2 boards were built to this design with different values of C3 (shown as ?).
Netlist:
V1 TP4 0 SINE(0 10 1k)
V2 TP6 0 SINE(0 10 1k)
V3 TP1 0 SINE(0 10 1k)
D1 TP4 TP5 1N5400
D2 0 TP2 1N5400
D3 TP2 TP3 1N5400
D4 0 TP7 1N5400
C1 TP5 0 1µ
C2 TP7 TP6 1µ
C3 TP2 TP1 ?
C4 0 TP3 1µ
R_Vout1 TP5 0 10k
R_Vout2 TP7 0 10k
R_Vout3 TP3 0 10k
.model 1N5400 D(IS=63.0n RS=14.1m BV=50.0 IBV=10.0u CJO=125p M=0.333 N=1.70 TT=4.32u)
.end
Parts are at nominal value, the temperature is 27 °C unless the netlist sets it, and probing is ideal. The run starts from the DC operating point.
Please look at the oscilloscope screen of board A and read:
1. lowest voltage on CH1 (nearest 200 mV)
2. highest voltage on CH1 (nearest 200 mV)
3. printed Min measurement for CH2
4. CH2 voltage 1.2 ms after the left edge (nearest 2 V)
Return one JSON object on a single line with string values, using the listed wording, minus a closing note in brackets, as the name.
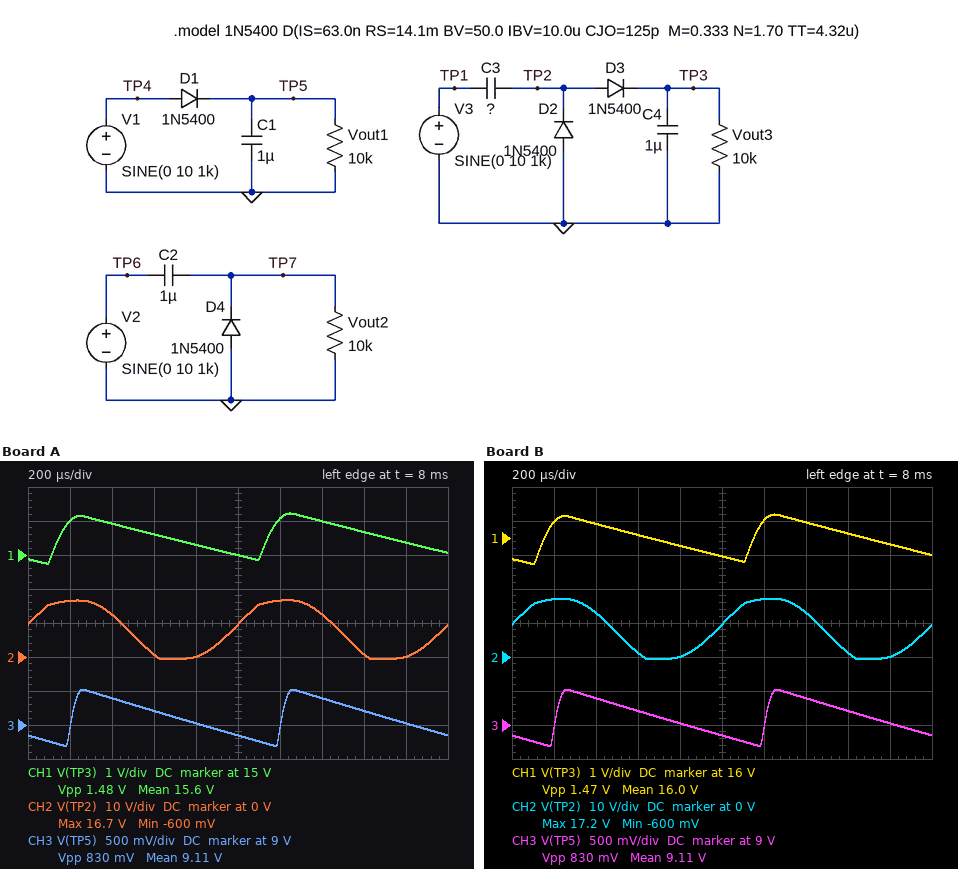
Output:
{"lowest voltage on CH1": "14.8 V", "highest voltage on CH1": "16.2 V", "printed Min measurement for CH2": "-600 mV", "CH2 voltage 1.2 ms after the left edge": "16 V"}
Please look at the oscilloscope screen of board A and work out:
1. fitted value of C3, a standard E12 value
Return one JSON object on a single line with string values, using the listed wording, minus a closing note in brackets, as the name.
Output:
{"fitted value of C3, a standard E12 value": "560 nF"}
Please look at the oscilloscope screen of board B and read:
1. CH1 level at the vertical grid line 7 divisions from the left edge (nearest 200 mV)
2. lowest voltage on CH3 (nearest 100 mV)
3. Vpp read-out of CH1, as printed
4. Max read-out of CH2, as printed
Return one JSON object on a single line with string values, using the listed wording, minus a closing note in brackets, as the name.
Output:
{"CH1 level at the vertical grid line 7 divisions from the left edge": "16.4 V", "lowest voltage on CH3": "8.7 V", "Vpp read-out of CH1, as printed": "1.47 V", "Max read-out of CH2, as printed": "17.2 V"}
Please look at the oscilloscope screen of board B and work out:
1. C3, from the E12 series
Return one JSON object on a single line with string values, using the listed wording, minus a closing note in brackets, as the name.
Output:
{"C3, from the E12 series": "680 nF"}
